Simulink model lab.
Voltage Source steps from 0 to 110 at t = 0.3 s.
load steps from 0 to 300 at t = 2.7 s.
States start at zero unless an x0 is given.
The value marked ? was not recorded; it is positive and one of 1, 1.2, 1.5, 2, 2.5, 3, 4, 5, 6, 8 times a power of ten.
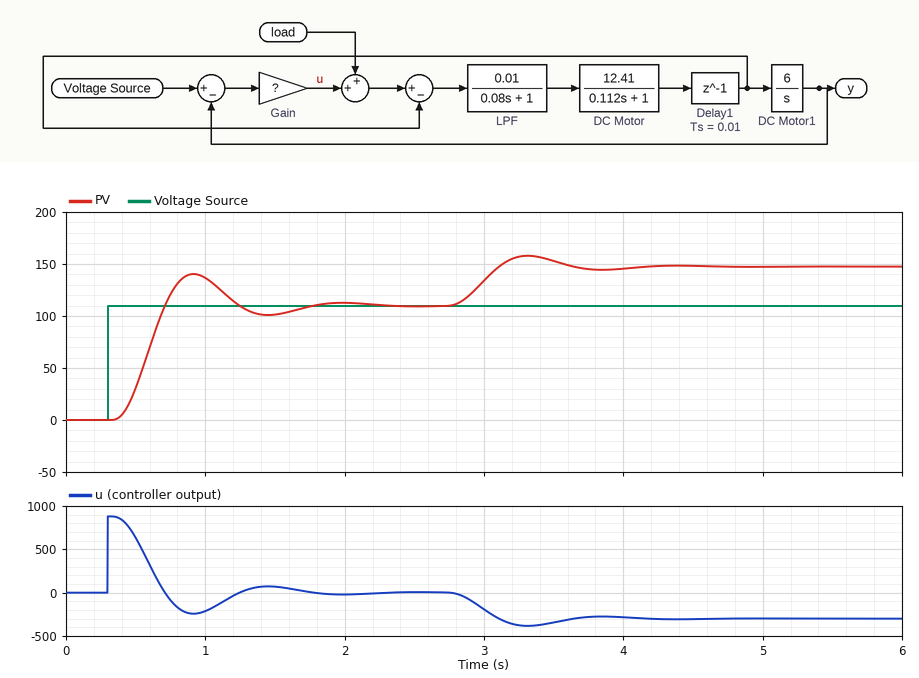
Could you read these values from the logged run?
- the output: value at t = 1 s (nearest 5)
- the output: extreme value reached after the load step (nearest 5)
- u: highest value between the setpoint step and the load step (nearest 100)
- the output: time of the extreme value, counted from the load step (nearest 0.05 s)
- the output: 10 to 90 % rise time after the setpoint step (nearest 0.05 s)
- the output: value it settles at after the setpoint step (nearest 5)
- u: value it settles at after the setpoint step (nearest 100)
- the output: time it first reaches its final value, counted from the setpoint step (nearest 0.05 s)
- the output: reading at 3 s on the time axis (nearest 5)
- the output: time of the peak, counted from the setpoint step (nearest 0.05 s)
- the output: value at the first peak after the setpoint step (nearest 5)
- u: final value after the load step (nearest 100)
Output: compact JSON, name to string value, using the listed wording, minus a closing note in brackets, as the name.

{"the output: value at t = 1 s": "135", "the output: extreme value reached after the load step": "160", "u: highest value between the setpoint step and the load step": "900", "the output: time of the extreme value, counted from the load step": "0.60 s", "the output: 10 to 90 % rise time after the setpoint step": "0.25 s", "the output: value it settles at after the setpoint step": "110", "u: value it settles at after the setpoint step": "0", "the output: time it first reaches its final value, counted from the setpoint step": "0.40 s", "the output: reading at 3 s on the time axis": "135", "the output: time of the peak, counted from the setpoint step": "0.60 s", "the output: value at the first peak after the setpoint step": "140", "u: final value after the load step": "-300"}
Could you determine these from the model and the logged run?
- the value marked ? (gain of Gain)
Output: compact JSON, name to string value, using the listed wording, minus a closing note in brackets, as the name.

{"the value marked ?": "8"}
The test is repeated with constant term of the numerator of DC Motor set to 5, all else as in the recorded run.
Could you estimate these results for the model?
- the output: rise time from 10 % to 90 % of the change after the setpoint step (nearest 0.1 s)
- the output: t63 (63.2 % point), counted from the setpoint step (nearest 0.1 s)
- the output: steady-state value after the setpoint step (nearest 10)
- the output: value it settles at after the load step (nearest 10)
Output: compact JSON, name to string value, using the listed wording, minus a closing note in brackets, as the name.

{"the output: rise time from 10 % to 90 % of the change after the setpoint step": "0.6 s", "the output: t63 (63.2 % point), counted from the setpoint step": "0.5 s", "the output: steady-state value after the setpoint step": "110", "the output: value it settles at after the load step": "150"}
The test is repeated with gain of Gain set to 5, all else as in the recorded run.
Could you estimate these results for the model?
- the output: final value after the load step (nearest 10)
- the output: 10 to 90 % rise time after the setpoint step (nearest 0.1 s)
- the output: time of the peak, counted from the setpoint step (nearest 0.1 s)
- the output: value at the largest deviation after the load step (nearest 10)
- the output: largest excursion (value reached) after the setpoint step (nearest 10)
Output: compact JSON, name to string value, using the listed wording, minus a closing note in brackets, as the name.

{"the output: final value after the load step": "170", "the output: 10 to 90 % rise time after the setpoint step": "0.4 s", "the output: time of the peak, counted from the setpoint step": "0.8 s", "the output: value at the largest deviation after the load step": "180", "the output: largest excursion (value reached) after the setpoint step": "120"}
